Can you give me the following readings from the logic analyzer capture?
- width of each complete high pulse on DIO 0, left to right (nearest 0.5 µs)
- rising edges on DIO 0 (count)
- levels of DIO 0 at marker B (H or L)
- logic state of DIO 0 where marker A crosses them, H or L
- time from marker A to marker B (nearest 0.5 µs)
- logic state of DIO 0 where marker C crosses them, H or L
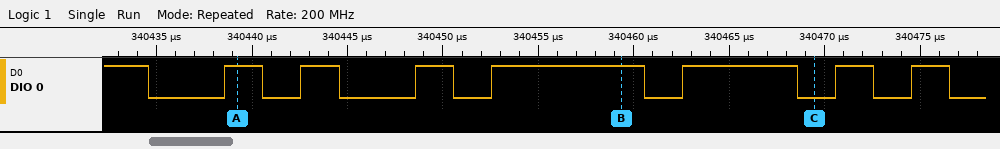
2 µs, 2 µs, 2 µs, 8 µs, 6 µs, 2 µs, 2 µs
7
DIO 0=H
DIO 0=H
20 µs
DIO 0=L
